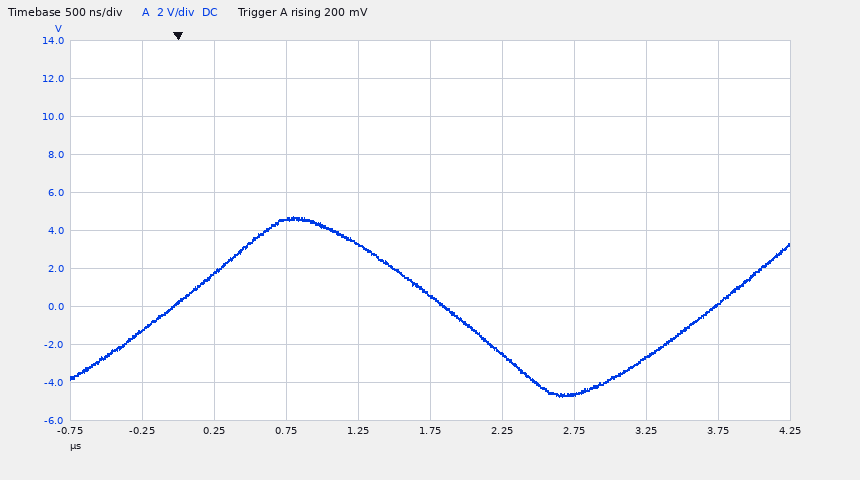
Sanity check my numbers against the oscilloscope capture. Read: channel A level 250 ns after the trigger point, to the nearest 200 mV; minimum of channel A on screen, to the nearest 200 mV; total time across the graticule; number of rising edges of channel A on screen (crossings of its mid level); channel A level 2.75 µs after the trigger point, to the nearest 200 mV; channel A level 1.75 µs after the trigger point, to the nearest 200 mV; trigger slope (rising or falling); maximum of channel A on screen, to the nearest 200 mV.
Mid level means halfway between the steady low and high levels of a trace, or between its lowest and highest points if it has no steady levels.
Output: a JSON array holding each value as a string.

["1.8 V", "-4.8 V", "5 µs", "2", "-4.6 V", "600 mV", "rising", "4.8 V"]
